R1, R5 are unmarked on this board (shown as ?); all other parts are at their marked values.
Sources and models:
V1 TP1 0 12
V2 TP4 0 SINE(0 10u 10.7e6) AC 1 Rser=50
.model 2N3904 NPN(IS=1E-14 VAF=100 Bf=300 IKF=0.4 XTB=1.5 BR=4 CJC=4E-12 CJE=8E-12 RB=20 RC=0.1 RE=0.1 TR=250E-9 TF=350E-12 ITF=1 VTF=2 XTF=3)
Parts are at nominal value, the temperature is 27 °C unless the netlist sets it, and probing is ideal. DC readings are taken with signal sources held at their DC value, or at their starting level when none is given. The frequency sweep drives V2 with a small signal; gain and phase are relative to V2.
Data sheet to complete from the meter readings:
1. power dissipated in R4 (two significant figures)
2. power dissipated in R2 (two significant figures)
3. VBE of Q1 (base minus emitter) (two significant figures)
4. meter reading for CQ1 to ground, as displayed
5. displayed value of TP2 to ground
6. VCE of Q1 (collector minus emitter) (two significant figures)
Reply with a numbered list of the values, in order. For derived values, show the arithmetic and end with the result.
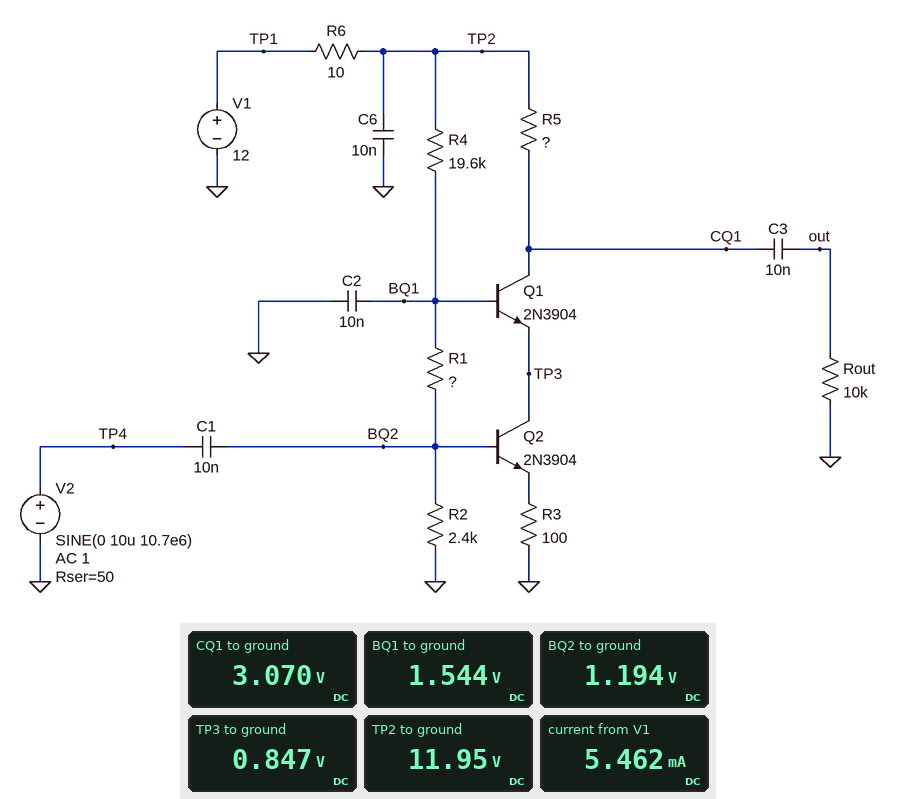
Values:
1. (11.95 V - 1.544 V)^2 / 19.6 kΩ = 5.5 mW
2. (1.194 V)^2 / 2.4 kΩ = 590 µW
3. 1.544 V - 847 mV = 700 mV
4. 3.070 V
5. 11.95 V
6. 3.07 V - 847 mV = 2.2 V
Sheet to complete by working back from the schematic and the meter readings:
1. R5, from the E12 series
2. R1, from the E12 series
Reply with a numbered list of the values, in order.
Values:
1. 1.8 kΩ
2. 680 Ω
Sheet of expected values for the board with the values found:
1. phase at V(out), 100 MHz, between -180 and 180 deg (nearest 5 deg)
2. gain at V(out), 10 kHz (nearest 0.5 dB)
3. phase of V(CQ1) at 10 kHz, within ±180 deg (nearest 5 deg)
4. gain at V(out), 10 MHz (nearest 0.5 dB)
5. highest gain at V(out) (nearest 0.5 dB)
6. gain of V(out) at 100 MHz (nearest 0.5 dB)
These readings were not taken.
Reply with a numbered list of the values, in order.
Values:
1. 40 deg
2. 16.5 dB
3. -150 deg
4. 22.0 dB
5. 22.5 dB
6. 12.5 dB
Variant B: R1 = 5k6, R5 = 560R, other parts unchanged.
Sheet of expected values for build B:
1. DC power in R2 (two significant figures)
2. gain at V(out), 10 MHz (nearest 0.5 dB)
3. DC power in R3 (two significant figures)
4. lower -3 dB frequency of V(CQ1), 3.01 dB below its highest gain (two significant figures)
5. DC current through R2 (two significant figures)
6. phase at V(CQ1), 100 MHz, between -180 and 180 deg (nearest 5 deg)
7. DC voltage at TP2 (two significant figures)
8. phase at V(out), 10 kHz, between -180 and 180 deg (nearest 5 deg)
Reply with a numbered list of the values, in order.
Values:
1. 420 µW
2. 13.5 dB
3. 1.0 mW
4. 10 kHz
5. 420 µA
6. 90 deg
7. 12 V
8. -130 deg
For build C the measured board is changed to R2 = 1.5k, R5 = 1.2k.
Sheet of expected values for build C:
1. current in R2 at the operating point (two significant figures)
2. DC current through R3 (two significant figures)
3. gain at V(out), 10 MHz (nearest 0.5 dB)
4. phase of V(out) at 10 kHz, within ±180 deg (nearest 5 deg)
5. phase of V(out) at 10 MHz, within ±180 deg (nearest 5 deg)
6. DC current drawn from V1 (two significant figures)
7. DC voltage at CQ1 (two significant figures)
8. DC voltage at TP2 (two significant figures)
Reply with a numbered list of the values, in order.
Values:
1. 540 µA
2. 1.5 mA
3. 18.0 dB
4. -130 deg
5. 165 deg
6. 2.0 mA
7. 10 V
8. 12 V
